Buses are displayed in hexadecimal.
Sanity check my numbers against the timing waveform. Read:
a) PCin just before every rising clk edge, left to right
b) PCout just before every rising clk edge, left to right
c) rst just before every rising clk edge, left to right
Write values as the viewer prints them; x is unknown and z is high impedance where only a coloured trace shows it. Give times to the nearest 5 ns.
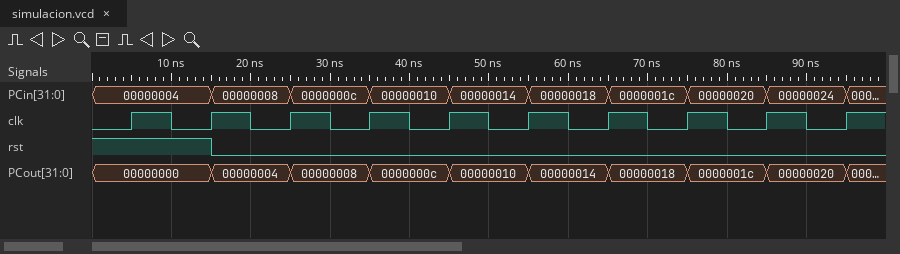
00000004, 00000004, 00000008, 0000000c, 00000010, 00000014, 00000018, 0000001c, 00000020, 00000024
00000000, 00000000, 00000004, 00000008, 0000000c, 00000010, 00000014, 00000018, 0000001c, 00000020
1 1 0 0 0 0 0 0 0 0
